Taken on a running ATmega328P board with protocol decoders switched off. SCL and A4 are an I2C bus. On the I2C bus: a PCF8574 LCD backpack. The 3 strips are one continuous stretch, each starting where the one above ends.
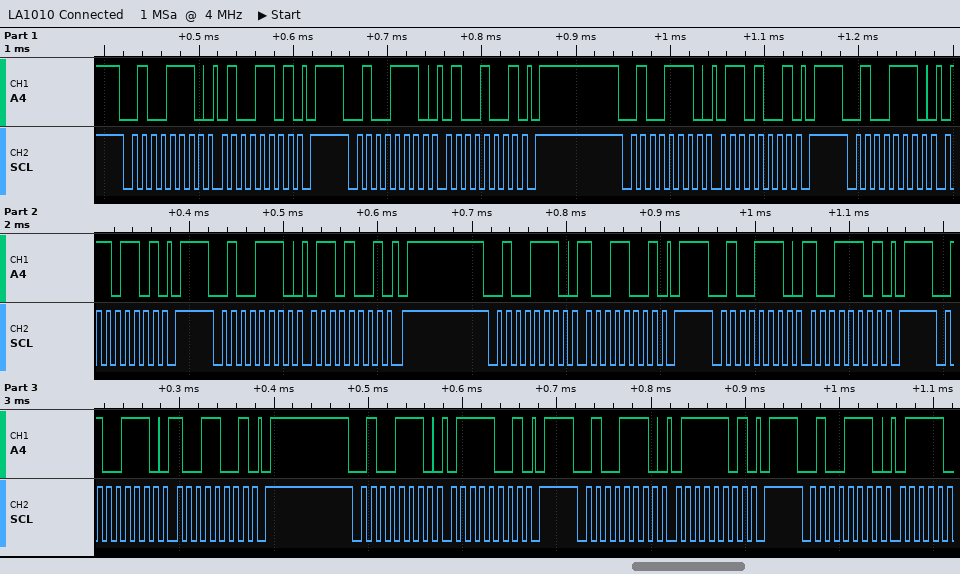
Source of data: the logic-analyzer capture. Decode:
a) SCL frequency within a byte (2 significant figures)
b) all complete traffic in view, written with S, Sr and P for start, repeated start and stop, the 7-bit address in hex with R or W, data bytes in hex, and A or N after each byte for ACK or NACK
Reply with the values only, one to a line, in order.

100 kHz
S 27W A 4D A P S 27W A 49 A P S 27W A 69 A P S 27W A 6D A P S 27W A 69 A P S 27W A 99 A P S 27W A 9D A P S 27W A 99 A P S 27W A 79 A P S 27W A 7D A P S 27W A
